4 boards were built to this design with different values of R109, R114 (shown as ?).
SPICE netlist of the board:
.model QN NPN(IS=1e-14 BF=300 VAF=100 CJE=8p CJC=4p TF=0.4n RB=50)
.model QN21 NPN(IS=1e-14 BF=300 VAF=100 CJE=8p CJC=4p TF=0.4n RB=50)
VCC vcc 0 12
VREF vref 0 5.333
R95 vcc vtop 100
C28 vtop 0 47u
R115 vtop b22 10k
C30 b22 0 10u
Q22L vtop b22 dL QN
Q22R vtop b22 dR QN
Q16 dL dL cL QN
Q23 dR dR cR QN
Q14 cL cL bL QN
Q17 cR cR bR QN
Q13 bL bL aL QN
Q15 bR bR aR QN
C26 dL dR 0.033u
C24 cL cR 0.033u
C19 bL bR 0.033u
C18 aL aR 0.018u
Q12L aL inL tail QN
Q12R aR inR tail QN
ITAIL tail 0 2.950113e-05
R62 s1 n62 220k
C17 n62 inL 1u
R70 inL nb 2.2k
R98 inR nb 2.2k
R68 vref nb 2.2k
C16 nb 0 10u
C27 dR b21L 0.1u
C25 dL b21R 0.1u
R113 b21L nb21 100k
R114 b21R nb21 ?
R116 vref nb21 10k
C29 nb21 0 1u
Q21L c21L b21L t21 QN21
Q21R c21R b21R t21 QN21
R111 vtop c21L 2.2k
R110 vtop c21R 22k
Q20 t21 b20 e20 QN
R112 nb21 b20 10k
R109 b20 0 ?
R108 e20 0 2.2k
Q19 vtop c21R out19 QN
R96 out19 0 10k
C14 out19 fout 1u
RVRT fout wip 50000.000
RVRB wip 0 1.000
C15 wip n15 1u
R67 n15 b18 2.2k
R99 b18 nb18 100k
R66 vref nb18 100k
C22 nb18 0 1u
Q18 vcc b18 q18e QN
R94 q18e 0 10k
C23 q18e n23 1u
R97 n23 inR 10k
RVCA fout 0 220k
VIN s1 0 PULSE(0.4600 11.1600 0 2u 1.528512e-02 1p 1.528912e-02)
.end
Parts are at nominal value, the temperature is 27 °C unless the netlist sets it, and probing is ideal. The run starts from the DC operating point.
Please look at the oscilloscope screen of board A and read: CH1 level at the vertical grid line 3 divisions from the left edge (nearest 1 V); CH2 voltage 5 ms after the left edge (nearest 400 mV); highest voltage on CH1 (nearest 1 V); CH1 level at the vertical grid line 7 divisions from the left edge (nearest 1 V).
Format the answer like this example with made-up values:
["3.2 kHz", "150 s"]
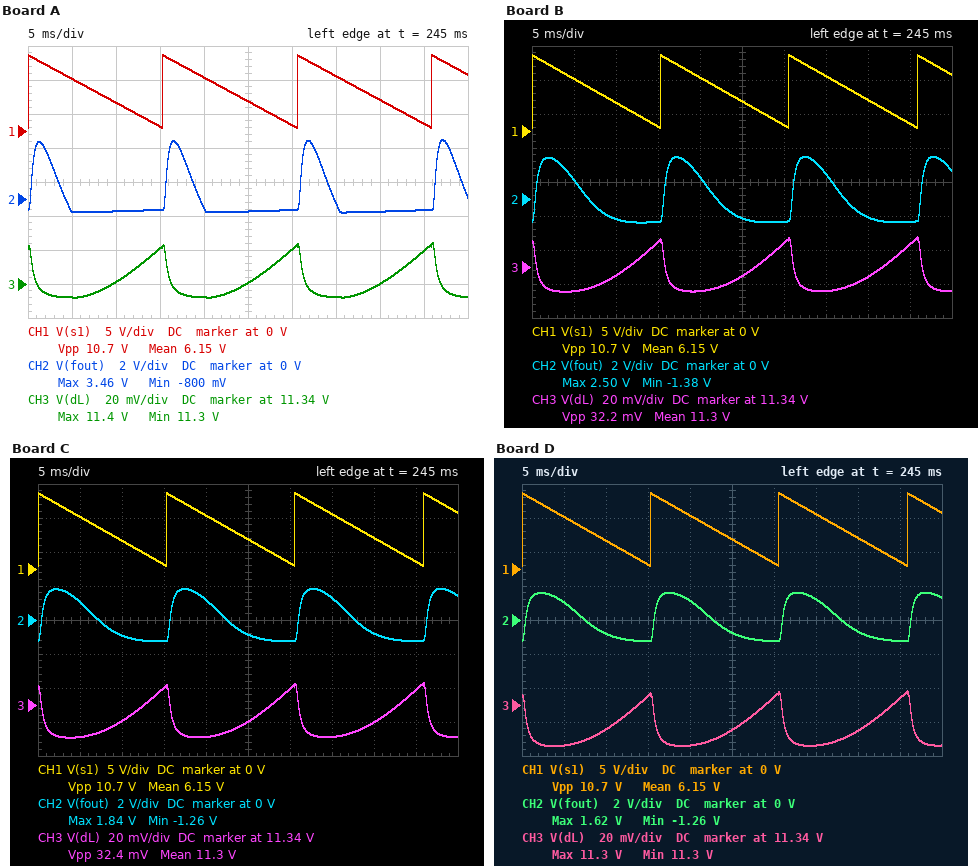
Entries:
["1 V", "-800 mV", "11 V", "8 V"]
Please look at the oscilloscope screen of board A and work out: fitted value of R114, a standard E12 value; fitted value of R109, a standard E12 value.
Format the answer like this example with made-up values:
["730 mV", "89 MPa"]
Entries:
["56 kΩ", "15 kΩ"]
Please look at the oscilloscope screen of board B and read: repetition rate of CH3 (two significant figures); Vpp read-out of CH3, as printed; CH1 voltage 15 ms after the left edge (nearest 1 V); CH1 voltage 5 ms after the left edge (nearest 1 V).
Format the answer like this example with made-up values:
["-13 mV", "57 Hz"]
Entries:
["66 Hz", "32.2 mV", "1 V", "8 V"]
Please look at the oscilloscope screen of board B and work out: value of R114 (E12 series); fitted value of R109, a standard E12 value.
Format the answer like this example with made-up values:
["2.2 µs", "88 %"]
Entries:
["120 kΩ", "8.2 kΩ"]
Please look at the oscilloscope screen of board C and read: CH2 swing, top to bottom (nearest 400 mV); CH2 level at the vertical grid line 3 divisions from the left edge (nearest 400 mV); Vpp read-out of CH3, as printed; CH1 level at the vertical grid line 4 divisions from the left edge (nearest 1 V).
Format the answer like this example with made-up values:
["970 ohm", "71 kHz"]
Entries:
["3.2 V", "-1.2 V", "32.4 mV", "8 V"]
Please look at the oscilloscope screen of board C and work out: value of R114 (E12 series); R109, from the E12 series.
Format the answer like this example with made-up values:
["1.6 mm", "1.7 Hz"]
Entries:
["180 kΩ", "6.8 kΩ"]
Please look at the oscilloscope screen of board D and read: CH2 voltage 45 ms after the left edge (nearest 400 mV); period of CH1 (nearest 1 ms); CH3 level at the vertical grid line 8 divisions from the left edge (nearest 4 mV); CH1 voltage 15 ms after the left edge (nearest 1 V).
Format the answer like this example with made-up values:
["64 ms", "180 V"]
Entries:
["-1.2 V", "15 ms", "11.324 V", "1 V"]
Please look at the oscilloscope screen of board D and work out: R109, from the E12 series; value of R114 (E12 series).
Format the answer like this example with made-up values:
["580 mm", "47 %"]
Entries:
["6.8 kΩ", "270 kΩ"]
